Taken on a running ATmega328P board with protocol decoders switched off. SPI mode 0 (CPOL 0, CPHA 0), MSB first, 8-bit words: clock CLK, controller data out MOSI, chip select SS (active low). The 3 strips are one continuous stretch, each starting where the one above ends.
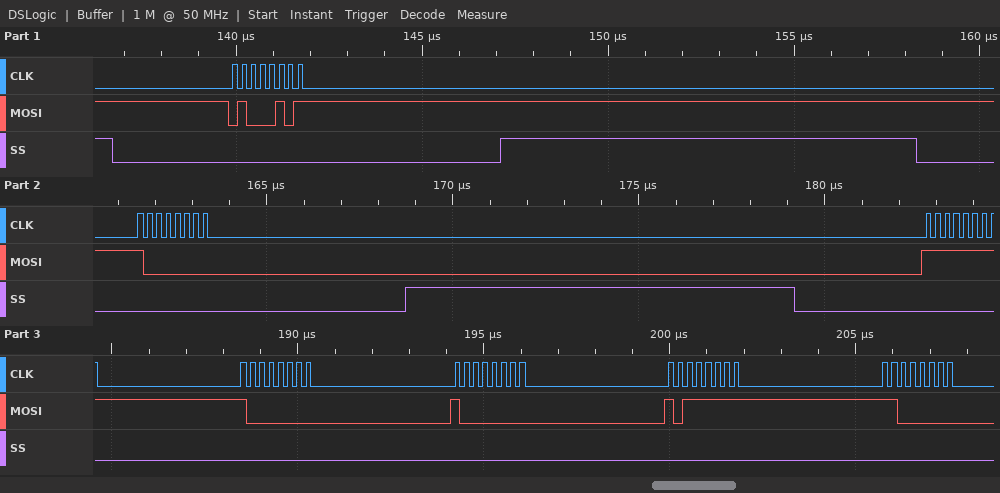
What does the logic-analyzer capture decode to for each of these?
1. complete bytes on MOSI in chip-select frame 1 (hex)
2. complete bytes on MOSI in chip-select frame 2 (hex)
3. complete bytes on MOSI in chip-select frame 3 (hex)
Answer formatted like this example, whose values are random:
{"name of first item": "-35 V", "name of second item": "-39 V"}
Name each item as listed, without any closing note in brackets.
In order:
{"complete bytes on MOSI in chip-select frame 1": "0x45", "complete bytes on MOSI in chip-select frame 2": "0x80", "complete bytes on MOSI in chip-select frame 3": "0xFF 0x80 0x80 0xBF 0xC0"}
